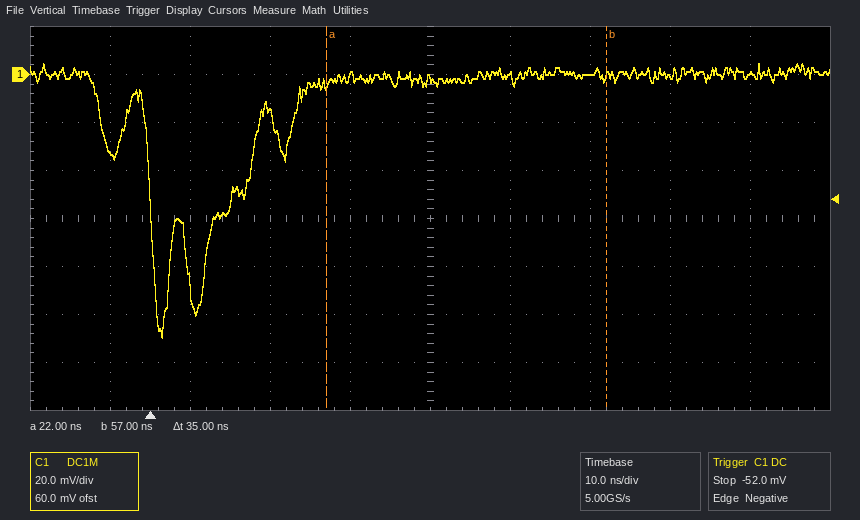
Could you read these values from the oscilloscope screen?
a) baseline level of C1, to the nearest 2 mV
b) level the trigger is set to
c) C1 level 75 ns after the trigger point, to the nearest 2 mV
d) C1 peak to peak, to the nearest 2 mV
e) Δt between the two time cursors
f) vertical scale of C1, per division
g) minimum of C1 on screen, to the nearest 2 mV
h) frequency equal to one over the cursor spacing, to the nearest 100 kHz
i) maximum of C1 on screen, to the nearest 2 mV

0 mV
-52.0 mV
0 mV
114 mV
35 ns
20 mV
-110 mV
28.6 MHz
4 mV
